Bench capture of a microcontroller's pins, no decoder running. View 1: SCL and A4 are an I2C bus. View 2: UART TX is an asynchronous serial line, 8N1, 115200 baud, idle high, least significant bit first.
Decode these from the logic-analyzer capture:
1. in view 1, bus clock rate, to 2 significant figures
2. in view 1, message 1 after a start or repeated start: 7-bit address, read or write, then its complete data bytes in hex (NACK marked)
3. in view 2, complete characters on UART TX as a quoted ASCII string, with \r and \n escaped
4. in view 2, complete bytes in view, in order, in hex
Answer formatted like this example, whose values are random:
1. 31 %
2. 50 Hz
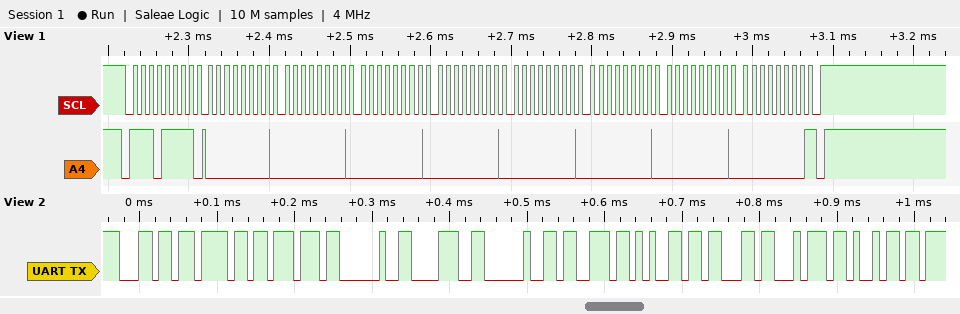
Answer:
1. 100 kHz
2. 0x77 read: 00 00 00 00 00 00 00 00 NACK
3. "low 8 secti"
4. 6C 6F 77 20 38 20 73 65 63 74 69
